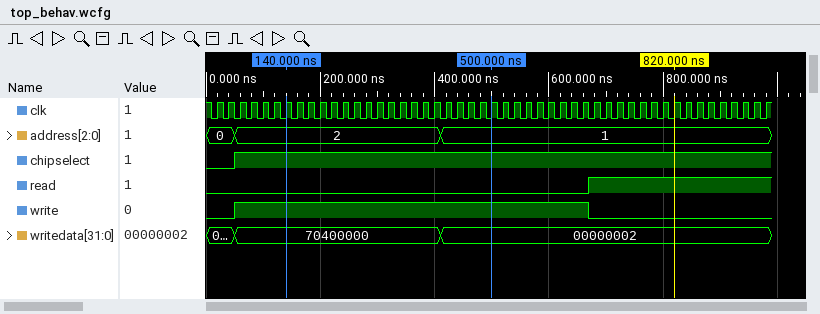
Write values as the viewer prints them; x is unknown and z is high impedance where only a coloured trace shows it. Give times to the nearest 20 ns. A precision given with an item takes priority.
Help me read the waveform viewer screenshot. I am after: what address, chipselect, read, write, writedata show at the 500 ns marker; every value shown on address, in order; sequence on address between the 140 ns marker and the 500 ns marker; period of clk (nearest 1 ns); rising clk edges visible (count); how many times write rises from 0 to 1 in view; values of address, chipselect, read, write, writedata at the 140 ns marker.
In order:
address=1, chipselect=1, read=0, write=1, writedata=00000002
0, 2, 1
2, 1
20 ns
49
1
address=2, chipselect=1, read=0, write=1, writedata=70400000
